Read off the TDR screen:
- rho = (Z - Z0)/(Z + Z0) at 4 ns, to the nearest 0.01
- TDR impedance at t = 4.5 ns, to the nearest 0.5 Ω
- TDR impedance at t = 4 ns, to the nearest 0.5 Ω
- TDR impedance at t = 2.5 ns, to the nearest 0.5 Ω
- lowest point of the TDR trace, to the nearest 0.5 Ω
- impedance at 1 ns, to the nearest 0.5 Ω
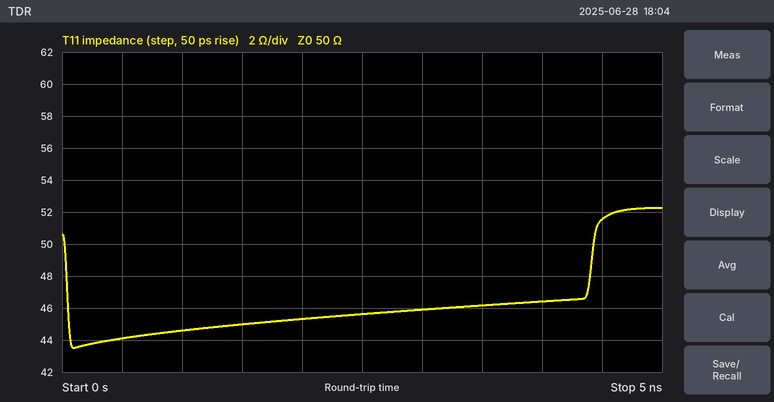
-0.04
51.5 Ω
46.5 Ω
45.5 Ω
43.5 Ω
44.5 Ω
